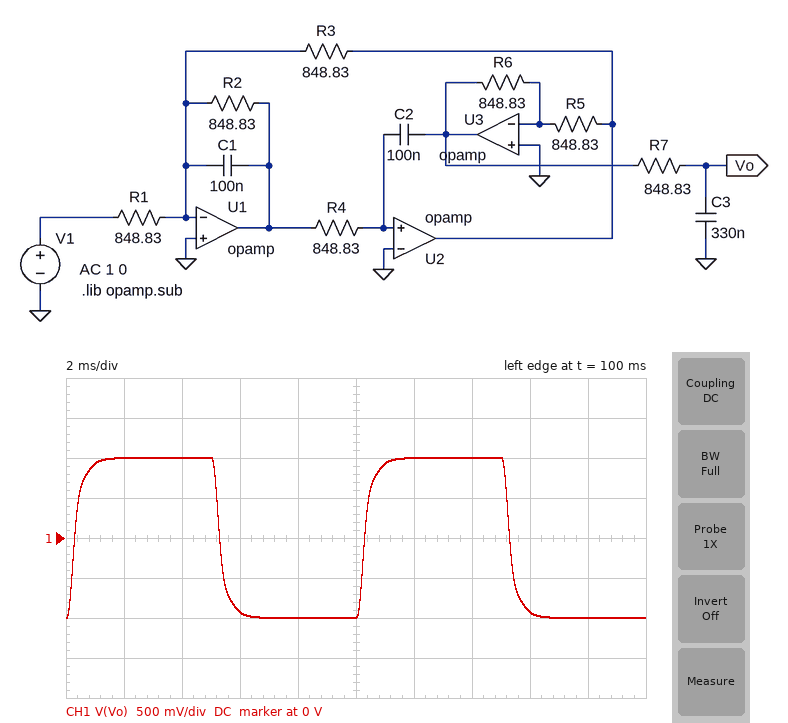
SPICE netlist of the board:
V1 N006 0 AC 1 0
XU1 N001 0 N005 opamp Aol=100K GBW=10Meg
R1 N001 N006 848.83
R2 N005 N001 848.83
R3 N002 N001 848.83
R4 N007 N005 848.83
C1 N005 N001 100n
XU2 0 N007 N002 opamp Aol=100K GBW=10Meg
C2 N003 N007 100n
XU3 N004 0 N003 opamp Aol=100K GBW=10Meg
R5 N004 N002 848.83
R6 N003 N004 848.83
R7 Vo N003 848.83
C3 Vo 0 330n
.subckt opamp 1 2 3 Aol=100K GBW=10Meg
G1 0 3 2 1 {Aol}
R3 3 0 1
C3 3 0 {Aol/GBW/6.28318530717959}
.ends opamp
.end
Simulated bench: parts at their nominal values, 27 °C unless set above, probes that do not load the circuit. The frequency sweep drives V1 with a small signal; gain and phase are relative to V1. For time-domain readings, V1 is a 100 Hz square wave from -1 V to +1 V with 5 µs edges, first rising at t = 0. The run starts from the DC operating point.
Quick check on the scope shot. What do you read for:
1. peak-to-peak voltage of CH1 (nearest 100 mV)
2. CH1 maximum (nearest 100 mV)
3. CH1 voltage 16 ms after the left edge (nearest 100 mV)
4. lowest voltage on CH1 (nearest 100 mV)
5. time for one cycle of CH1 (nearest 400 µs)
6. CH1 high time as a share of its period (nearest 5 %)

2.0 V
1.0 V
-900 mV
-1.0 V
10.0 ms
50 %
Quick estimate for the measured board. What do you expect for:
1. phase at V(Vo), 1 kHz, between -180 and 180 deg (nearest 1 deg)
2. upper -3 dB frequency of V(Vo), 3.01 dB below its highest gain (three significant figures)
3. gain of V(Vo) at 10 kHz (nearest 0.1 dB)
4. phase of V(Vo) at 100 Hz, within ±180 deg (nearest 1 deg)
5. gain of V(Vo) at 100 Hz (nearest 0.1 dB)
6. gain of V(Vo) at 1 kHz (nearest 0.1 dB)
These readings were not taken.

-97 deg
628 Hz
-53.9 dB
-13 deg
-0.1 dB
-5.1 dB
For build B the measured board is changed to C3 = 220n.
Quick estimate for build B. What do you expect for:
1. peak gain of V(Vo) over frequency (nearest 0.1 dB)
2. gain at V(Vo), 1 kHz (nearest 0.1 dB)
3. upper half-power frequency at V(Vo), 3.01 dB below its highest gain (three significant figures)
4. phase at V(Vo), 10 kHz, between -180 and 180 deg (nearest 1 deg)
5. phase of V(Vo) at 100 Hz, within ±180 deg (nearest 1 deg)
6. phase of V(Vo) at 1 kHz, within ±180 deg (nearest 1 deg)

0 dB
-2.8 dB
1.06 kHz
106 deg
-10 deg
-86 deg
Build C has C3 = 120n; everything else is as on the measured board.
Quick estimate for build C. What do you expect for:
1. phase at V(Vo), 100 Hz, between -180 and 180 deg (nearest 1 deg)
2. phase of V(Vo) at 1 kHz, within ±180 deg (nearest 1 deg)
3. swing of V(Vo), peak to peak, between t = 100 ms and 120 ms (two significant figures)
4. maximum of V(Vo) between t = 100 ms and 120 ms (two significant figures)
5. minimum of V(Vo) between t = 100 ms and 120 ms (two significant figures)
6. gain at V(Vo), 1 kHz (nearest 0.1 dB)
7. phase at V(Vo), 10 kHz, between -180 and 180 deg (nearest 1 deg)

-7 deg
-69 deg
2.2 V
1.1 V
-1.1 V
-0.5 dB
110 deg
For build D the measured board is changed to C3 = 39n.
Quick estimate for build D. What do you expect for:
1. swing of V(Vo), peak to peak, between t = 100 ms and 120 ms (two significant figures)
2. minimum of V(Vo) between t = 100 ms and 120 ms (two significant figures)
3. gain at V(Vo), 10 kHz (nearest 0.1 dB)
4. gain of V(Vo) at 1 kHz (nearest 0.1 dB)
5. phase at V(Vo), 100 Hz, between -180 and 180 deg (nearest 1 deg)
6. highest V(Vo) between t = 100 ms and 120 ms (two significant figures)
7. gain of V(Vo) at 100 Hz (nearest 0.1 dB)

2.6 V
-1.3 V
-36.2 dB
0.8 dB
-4 deg
1.3 V
0 dB
